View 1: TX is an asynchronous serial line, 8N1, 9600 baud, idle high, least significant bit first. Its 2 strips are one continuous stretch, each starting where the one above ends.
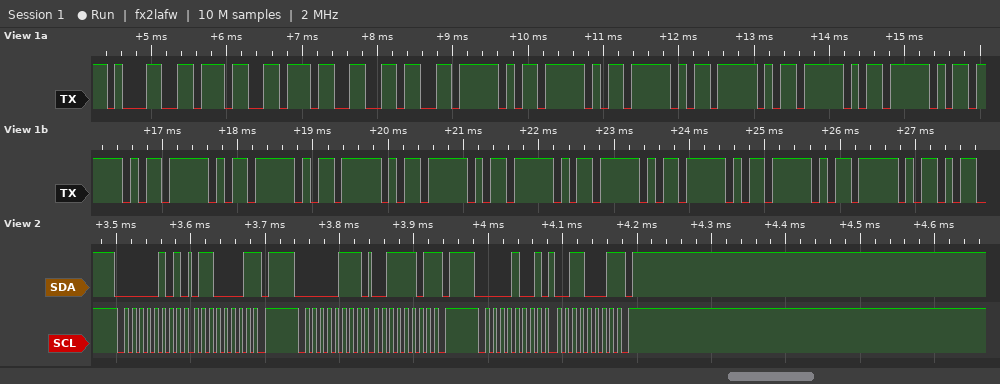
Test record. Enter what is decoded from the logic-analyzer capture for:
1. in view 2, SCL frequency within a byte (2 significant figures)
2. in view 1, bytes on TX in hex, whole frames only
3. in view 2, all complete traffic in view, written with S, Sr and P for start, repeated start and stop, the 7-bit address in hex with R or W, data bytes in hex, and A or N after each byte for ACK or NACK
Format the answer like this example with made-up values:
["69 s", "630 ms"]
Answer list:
["100 kHz", "31 37 37 36 5F 5F 5F 5F 5F 5F 5F 5F 5F 5F 5F 5F 5F 5F 5F 5F", "S 02R A 61 N P S 03R A 3D N P S 04R A 31 N P"]
